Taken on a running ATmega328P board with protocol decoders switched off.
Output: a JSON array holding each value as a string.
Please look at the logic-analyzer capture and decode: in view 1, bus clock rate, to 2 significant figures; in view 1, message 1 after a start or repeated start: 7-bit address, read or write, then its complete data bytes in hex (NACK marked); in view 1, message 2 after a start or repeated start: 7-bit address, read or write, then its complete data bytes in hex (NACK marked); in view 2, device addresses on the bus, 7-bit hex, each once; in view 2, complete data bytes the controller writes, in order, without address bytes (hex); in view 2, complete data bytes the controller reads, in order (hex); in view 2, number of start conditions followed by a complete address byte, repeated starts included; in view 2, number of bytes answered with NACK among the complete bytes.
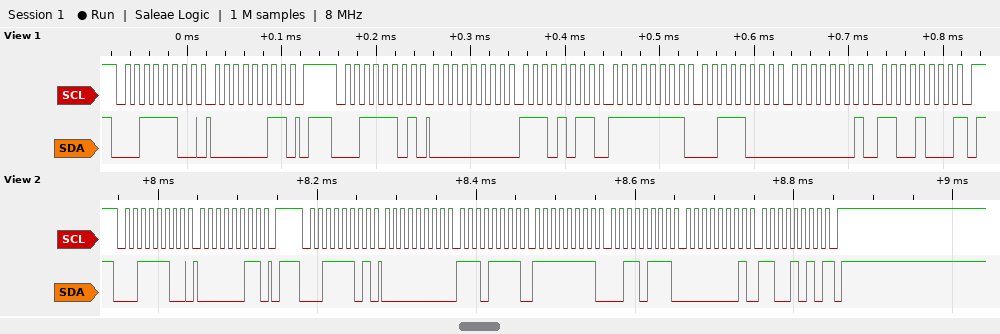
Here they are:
["100 kHz", "0x1E write: 03", "0x1E read: 00 EB FF 38 01 C8 NACK", "0x1E", "03", "00 EF FF 37 01 CA", "2", "1"]
